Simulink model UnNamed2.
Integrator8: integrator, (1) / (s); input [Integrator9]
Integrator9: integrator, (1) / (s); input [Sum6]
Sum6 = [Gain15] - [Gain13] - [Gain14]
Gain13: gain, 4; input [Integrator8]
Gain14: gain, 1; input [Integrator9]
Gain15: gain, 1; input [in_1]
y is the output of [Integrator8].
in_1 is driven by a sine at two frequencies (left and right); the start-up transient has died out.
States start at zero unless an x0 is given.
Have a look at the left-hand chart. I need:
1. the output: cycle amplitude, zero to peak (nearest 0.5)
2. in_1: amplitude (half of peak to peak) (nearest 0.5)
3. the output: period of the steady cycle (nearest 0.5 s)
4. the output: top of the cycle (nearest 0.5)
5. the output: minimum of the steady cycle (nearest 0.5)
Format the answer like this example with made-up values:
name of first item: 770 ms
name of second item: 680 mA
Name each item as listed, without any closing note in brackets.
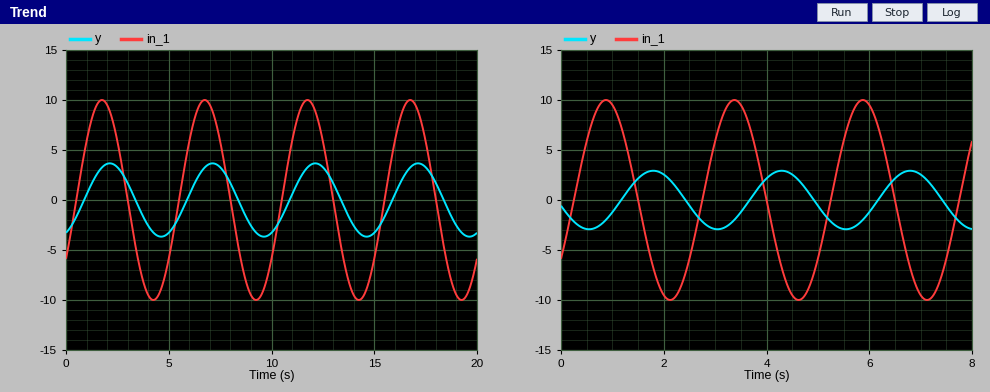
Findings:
the output: cycle amplitude, zero to peak: 3.5
in_1: amplitude (half of peak to peak): 10.0
the output: period of the steady cycle: 5.0 s
the output: top of the cycle: 3.5
the output: minimum of the steady cycle: -3.5
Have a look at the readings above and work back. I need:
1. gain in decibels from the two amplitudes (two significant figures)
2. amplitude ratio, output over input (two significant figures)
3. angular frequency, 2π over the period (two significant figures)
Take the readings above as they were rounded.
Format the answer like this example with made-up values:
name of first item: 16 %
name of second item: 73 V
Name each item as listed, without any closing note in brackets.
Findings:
gain in decibels from the two amplitudes: -9.1 dB
amplitude ratio, output over input: 0.35
angular frequency, 2π over the period: 1.3 rad/s
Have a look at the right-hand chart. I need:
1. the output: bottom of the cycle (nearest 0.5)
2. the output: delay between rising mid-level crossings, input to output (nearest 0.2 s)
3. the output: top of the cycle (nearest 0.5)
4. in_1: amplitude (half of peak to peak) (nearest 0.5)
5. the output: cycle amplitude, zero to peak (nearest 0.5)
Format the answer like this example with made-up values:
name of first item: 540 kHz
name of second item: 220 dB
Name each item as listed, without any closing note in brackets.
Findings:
the output: bottom of the cycle: -3.0
the output: delay between rising mid-level crossings, input to output: 1.0 s
the output: top of the cycle: 3.0
in_1: amplitude (half of peak to peak): 10.0
the output: cycle amplitude, zero to peak: 3.0
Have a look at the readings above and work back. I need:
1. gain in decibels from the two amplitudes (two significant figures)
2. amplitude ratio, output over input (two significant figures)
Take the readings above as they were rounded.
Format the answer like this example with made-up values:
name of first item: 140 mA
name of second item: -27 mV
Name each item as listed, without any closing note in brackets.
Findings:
gain in decibels from the two amplitudes: -10 dB
amplitude ratio, output over input: 0.30
